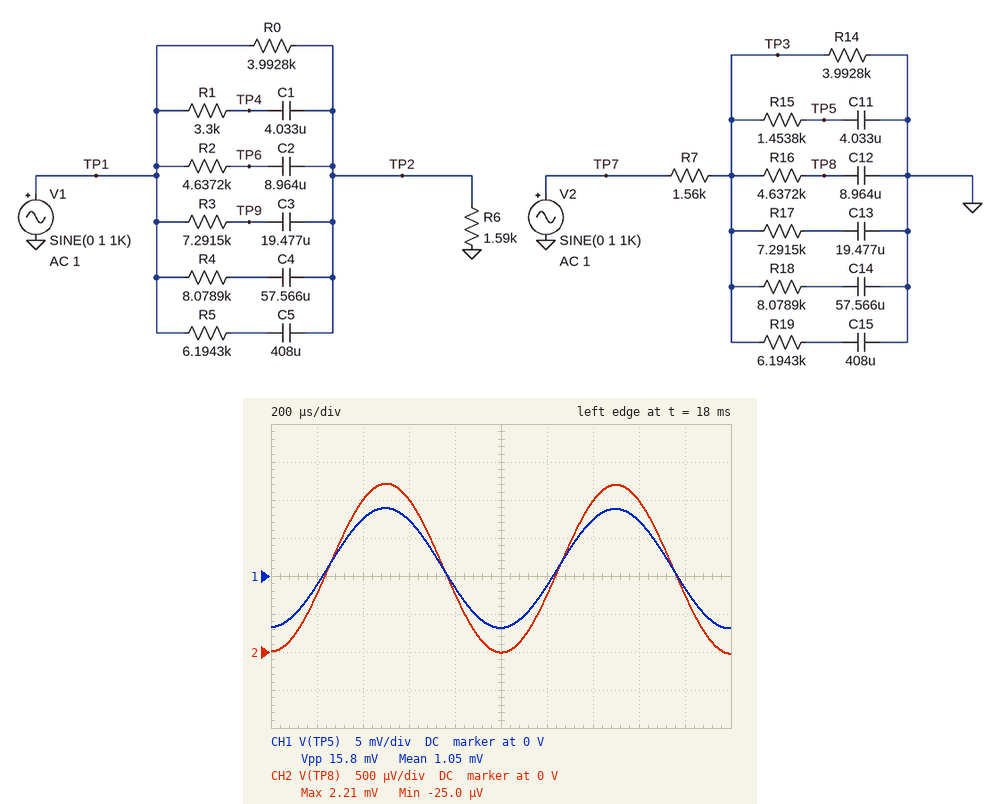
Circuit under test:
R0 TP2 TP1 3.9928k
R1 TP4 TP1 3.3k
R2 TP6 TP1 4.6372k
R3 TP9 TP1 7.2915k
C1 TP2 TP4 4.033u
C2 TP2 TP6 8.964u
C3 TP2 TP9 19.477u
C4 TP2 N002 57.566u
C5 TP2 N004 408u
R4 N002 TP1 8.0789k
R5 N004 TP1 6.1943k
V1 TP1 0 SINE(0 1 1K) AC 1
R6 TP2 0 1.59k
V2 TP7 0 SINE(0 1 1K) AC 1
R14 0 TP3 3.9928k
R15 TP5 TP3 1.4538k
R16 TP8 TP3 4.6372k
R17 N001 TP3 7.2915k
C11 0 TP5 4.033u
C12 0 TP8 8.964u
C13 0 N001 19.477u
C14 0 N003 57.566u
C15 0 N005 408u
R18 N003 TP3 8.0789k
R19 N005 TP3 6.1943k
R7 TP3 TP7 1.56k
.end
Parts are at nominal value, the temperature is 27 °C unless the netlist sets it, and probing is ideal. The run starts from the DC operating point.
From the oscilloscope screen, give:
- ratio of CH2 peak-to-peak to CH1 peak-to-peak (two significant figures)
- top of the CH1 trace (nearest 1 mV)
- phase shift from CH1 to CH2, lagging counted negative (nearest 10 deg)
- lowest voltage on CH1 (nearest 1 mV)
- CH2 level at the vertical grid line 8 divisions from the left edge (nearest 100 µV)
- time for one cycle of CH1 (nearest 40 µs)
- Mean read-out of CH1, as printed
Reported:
0.14
9 mV
0 deg
-7 mV
2.0 mV
1.00 ms
1.05 mV
